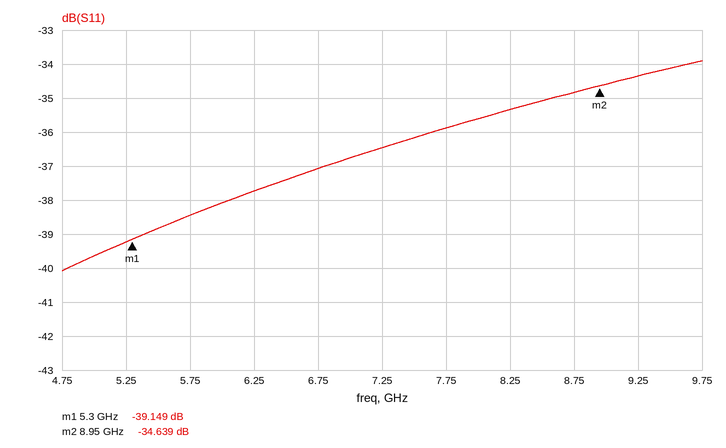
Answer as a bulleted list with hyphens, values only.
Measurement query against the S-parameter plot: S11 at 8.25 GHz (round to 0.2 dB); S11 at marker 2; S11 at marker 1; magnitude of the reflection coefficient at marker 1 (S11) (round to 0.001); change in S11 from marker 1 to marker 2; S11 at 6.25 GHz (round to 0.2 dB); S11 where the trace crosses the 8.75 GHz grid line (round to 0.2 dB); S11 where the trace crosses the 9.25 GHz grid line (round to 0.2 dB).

- -35.4 dB
- -34.639 dB
- -39.149 dB
- 0.011
- 4.510 dB
- -37.8 dB
- -34.8 dB
- -34.4 dB
